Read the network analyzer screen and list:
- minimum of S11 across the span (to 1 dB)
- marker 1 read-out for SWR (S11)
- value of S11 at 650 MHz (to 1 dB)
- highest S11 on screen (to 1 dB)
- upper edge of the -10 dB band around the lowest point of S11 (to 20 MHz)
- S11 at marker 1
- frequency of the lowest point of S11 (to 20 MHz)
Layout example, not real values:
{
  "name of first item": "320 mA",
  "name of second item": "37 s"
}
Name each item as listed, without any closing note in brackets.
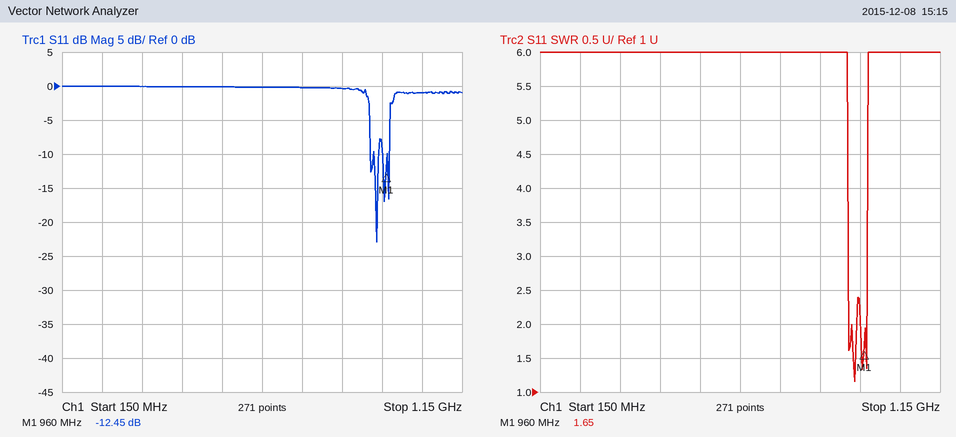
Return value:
{
  "minimum of S11 across the span": "-23 dB",
  "marker 1 read-out for SWR": "1.65",
  "value of S11 at 650 MHz": "0 dB",
  "highest S11 on screen": "0 dB",
  "upper edge of the -10 dB band around the lowest point of S11": "940 MHz",
  "S11 at marker 1": "-12.45 dB",
  "frequency of the lowest point of S11": "940 MHz"
}
